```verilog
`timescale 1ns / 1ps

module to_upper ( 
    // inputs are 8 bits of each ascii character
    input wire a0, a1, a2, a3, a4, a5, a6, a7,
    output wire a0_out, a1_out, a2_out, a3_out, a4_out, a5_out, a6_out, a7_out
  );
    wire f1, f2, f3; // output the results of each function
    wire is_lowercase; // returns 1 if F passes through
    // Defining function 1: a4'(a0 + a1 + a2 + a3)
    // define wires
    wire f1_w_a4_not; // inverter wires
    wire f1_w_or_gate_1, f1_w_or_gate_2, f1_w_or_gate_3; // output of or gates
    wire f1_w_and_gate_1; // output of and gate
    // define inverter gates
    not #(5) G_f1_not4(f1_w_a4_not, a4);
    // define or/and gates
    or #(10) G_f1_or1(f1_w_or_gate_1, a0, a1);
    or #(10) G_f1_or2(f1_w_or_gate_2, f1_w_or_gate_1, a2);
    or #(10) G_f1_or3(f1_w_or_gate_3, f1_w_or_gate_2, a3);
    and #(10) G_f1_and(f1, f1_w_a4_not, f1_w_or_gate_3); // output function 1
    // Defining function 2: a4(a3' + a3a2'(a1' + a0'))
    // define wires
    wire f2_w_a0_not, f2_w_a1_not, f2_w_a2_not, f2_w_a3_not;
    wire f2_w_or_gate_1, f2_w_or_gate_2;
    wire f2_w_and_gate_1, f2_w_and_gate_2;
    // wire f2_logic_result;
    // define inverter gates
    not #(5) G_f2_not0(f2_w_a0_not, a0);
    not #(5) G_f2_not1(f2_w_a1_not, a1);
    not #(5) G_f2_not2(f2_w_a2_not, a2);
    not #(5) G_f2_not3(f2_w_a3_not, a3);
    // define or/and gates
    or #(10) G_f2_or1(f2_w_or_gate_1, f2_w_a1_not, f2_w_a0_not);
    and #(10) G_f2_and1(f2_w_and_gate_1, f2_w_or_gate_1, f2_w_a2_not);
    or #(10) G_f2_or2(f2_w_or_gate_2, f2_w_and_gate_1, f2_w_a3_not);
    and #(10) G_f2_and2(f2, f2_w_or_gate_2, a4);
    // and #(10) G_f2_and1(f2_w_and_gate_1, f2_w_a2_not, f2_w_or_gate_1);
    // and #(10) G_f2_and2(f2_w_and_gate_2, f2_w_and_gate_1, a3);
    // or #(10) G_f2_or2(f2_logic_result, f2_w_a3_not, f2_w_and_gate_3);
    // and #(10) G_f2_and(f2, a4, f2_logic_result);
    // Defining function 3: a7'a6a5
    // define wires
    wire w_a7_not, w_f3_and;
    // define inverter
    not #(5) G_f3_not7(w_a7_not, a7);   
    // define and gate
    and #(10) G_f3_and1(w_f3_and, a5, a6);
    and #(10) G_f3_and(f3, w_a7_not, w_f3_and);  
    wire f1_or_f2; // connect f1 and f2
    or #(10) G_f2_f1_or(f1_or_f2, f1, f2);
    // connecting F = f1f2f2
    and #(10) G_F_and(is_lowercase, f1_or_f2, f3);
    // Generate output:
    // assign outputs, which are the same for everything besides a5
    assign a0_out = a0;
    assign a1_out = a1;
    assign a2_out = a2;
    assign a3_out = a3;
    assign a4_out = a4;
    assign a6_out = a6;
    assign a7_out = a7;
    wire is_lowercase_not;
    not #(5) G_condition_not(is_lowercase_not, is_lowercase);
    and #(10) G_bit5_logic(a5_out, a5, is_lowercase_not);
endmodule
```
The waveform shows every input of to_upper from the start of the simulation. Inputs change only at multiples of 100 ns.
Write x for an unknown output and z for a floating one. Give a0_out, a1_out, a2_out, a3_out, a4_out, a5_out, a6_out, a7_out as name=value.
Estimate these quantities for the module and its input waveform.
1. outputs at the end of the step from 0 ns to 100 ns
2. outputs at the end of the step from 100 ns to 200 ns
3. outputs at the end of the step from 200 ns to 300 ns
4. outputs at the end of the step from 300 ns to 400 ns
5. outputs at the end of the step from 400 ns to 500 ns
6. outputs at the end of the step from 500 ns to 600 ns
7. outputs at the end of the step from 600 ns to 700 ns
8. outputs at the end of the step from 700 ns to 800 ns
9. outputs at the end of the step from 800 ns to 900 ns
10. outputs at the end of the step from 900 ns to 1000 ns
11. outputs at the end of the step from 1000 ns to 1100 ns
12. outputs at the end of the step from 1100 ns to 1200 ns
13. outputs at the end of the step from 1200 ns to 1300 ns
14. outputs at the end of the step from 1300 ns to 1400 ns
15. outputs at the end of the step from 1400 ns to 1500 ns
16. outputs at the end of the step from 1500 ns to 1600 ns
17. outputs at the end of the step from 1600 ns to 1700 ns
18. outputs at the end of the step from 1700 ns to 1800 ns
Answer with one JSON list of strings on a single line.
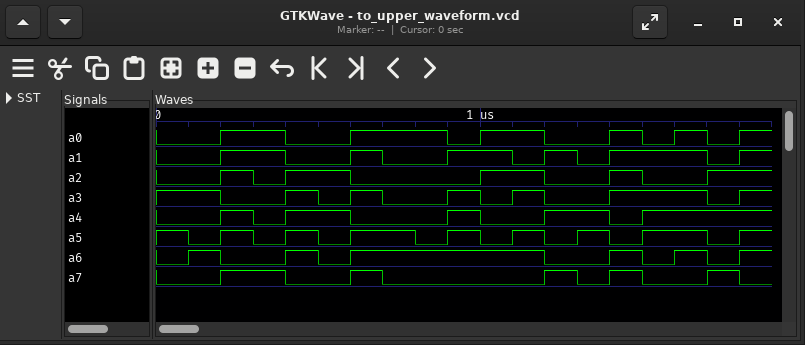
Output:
["a0_out=0, a1_out=0, a2_out=0, a3_out=1, a4_out=0, a5_out=1, a6_out=0, a7_out=0", "a0_out=0, a1_out=0, a2_out=0, a3_out=1, a4_out=0, a5_out=0, a6_out=1, a7_out=0", "a0_out=1, a1_out=1, a2_out=1, a3_out=0, a4_out=1, a5_out=1, a6_out=0, a7_out=1", "a0_out=1, a1_out=1, a2_out=0, a3_out=0, a4_out=0, a5_out=0, a6_out=0, a7_out=1", "a0_out=0, a1_out=0, a2_out=1, a3_out=1, a4_out=1, a5_out=1, a6_out=1, a7_out=0", "a0_out=0, a1_out=0, a2_out=1, a3_out=0, a4_out=1, a5_out=0, a6_out=0, a7_out=0", "a0_out=1, a1_out=1, a2_out=0, a3_out=1, a4_out=0, a5_out=1, a6_out=1, a7_out=1", "a0_out=1, a1_out=0, a2_out=0, a3_out=0, a4_out=0, a5_out=0, a6_out=1, a7_out=0", "a0_out=1, a1_out=0, a2_out=0, a3_out=0, a4_out=0, a5_out=0, a6_out=1, a7_out=0", "a0_out=0, a1_out=1, a2_out=0, a3_out=1, a4_out=1, a5_out=0, a6_out=1, a7_out=0", "a0_out=1, a1_out=1, a2_out=1, a3_out=0, a4_out=0, a5_out=0, a6_out=1, a7_out=0", "a0_out=1, a1_out=0, a2_out=1, a3_out=1, a4_out=0, a5_out=0, a6_out=1, a7_out=0", "a0_out=0, a1_out=1, a2_out=0, a3_out=0, a4_out=1, a5_out=0, a6_out=0, a7_out=1", "a0_out=0, a1_out=0, a2_out=0, a3_out=0, a4_out=1, a5_out=1, a6_out=0, a7_out=0", "a0_out=1, a1_out=1, a2_out=1, a3_out=1, a4_out=0, a5_out=0, a6_out=1, a7_out=1", "a0_out=0, a1_out=1, a2_out=0, a3_out=1, a4_out=1, a5_out=1, a6_out=0, a7_out=0", "a0_out=1, a1_out=1, a2_out=0, a3_out=1, a4_out=1, a5_out=1, a6_out=1, a7_out=0", "a0_out=0, a1_out=0, a2_out=1, a3_out=0, a4_out=1, a5_out=0, a6_out=0, a7_out=1"]
